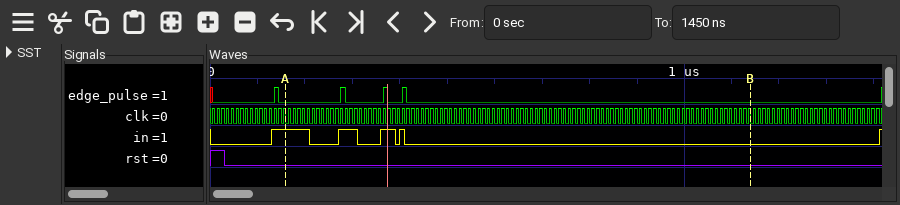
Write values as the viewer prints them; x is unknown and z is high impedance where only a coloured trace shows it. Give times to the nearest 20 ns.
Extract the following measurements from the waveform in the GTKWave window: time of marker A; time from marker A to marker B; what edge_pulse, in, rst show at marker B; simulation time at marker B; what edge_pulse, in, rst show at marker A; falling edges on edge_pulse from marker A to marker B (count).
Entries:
160 ns
980 ns
edge_pulse=0, in=0, rst=0
1140 ns
edge_pulse=0, in=1, rst=0
3
